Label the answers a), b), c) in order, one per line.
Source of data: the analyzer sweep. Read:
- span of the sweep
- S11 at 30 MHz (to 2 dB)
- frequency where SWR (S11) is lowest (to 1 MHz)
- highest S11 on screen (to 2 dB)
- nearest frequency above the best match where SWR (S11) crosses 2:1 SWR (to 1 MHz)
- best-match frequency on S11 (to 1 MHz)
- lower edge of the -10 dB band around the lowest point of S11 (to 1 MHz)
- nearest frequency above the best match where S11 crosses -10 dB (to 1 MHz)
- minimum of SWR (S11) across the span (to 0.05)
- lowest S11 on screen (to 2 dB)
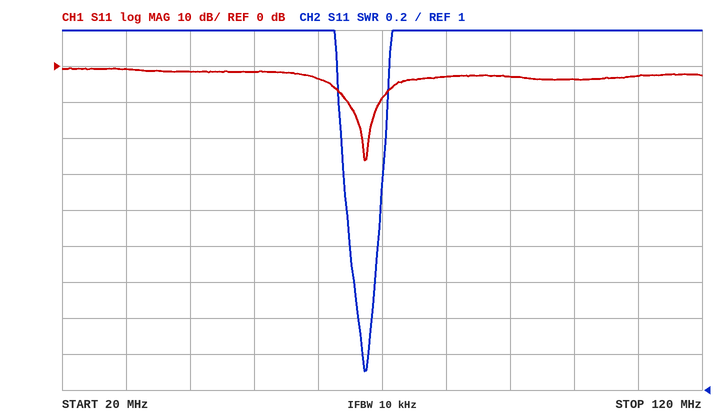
a) 100 MHz
b) 0 dB
c) 67 MHz
d) 0 dB
e) 70 MHz
f) 67 MHz
g) 65 MHz
h) 70 MHz
i) 1.10
j) -26 dB
